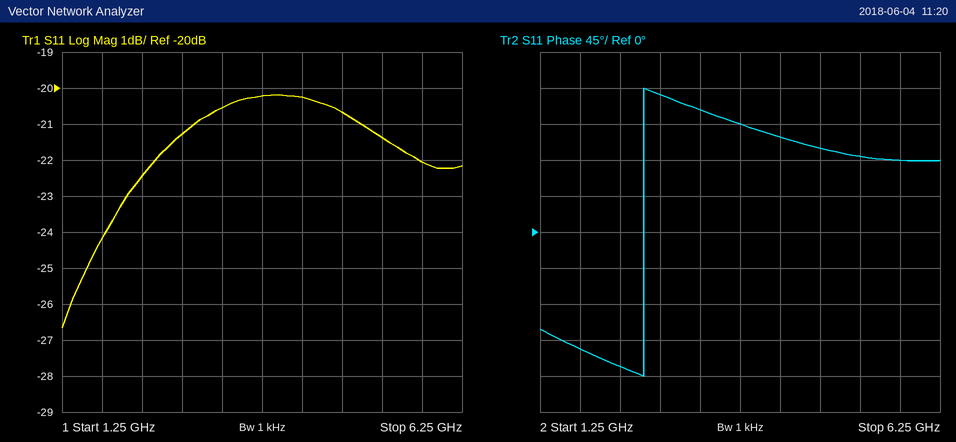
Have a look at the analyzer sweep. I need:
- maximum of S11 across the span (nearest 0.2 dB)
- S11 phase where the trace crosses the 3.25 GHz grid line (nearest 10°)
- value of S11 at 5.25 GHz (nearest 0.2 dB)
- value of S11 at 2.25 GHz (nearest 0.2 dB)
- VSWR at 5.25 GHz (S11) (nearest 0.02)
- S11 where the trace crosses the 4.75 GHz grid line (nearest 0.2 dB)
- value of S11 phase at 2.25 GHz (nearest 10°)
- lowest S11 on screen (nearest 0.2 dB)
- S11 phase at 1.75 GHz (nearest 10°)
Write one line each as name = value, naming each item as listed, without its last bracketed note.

maximum of S11 across the span = -20.2 dB
S11 phase where the trace crosses the 3.25 GHz grid line = 150°
value of S11 at 5.25 GHz = -21.4 dB
value of S11 at 2.25 GHz = -22.4 dB
VSWR at 5.25 GHz (S11) = 1.18
S11 where the trace crosses the 4.75 GHz grid line = -20.6 dB
value of S11 phase at 2.25 GHz = -170°
lowest S11 on screen = -26.6 dB
S11 phase at 1.75 GHz = -150°
